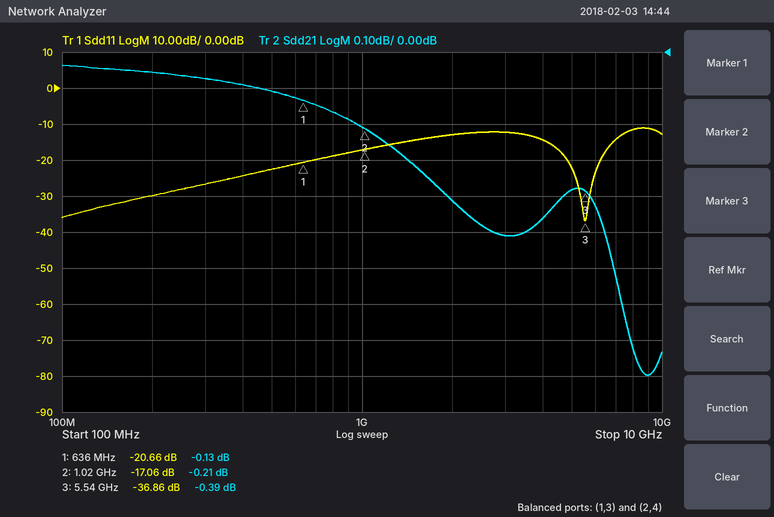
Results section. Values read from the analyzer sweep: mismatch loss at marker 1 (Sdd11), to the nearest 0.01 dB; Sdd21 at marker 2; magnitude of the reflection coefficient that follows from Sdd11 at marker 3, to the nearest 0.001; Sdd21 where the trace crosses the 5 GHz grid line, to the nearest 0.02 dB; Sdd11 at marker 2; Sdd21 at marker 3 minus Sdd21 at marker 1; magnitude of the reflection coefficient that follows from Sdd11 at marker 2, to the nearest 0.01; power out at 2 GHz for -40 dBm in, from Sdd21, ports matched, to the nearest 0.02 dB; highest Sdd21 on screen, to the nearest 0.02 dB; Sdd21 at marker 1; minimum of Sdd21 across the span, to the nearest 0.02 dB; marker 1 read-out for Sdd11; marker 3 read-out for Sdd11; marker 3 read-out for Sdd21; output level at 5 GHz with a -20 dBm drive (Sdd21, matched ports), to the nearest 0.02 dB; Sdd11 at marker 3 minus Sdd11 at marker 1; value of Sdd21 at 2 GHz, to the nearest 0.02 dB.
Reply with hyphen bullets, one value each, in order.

- 0.04 dB
- -0.21 dB
- 0.014
- -0.38 dB
- -17.06 dB
- -0.26 dB
- 0.14
- -40.42 dBm
- -0.04 dB
- -0.13 dB
- -0.90 dB
- -20.66 dB
- -36.86 dB
- -0.39 dB
- -20.38 dBm
- -16.20 dB
- -0.42 dB
